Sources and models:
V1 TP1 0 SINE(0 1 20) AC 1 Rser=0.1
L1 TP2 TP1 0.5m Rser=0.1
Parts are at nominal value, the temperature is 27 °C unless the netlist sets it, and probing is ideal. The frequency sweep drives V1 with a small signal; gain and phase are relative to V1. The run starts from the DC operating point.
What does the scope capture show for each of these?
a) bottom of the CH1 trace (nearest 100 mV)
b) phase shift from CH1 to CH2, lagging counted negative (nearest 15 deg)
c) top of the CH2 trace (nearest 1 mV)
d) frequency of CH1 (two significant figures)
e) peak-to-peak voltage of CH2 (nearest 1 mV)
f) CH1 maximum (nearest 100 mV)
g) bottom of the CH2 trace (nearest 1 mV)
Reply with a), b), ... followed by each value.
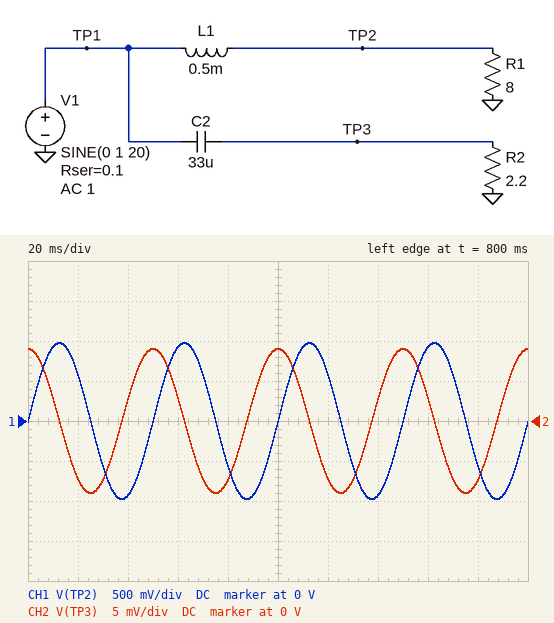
a) -1.0 V
b) 90 deg
c) 9 mV
d) 20 Hz
e) 18 mV
f) 1.0 V
g) -9 mV
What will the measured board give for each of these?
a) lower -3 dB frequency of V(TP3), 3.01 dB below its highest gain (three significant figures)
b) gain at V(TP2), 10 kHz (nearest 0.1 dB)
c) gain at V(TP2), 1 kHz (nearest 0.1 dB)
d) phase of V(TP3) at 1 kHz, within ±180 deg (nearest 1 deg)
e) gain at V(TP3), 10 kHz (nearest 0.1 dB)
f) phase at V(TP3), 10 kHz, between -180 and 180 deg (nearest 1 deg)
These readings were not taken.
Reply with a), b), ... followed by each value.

a) 2.13 kHz
b) -12.5 dB
c) -0.9 dB
d) 65 deg
e) -0.6 dB
f) 12 deg
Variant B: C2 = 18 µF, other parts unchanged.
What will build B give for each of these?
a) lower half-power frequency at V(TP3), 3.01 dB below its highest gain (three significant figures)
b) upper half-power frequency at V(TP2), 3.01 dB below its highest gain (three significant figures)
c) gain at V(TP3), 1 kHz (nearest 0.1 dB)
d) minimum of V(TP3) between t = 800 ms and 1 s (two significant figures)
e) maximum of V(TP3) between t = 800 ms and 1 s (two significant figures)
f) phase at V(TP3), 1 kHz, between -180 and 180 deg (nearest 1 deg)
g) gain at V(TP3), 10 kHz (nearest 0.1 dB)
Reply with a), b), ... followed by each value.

a) 3.87 kHz
b) 2.54 kHz
c) -12.5 dB
d) -4.9 mV
e) 4.9 mV
f) 76 deg
g) -1.0 dB
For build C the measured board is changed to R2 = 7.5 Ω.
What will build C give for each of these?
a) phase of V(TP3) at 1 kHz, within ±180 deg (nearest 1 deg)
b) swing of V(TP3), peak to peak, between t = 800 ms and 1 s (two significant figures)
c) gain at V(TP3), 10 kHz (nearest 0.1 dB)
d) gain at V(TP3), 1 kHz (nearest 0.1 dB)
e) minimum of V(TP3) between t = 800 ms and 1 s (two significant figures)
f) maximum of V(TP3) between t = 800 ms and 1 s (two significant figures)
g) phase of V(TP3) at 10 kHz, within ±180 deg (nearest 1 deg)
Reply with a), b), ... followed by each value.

a) 33 deg
b) 61 mV
c) -0.1 dB
d) -1.7 dB
e) -31 mV
f) 31 mV
g) 4 deg
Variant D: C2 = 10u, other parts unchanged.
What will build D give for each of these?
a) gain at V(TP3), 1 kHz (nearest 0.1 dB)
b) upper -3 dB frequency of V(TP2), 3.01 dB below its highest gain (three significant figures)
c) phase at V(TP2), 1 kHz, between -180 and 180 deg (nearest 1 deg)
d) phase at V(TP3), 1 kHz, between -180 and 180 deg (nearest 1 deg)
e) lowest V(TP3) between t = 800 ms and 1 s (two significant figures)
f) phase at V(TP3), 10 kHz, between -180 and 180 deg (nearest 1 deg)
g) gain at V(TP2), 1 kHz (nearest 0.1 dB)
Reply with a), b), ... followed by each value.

a) -17.4 dB
b) 2.58 kHz
c) -21 deg
d) 82 deg
e) -2.7 mV
f) 35 deg
g) -0.8 dB
